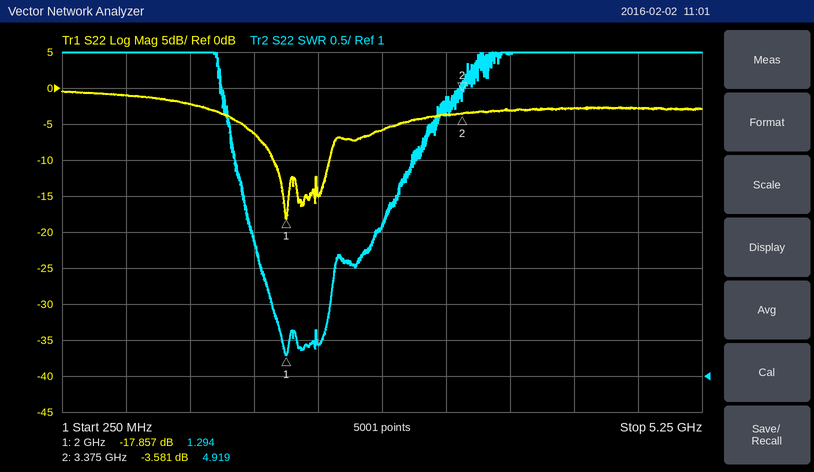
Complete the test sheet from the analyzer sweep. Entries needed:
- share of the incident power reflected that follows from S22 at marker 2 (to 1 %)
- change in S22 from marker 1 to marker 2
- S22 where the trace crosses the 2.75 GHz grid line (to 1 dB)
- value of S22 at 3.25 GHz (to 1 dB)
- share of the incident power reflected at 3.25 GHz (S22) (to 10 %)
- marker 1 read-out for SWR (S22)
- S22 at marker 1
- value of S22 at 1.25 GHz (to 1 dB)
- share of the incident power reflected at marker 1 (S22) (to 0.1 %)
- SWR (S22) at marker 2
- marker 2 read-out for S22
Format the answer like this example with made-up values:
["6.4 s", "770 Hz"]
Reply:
["44 %", "14.276 dB", "-6 dB", "-4 dB", "40 %", "1.294", "-17.857 dB", "-2 dB", "1.6 %", "4.919", "-3.581 dB"]
